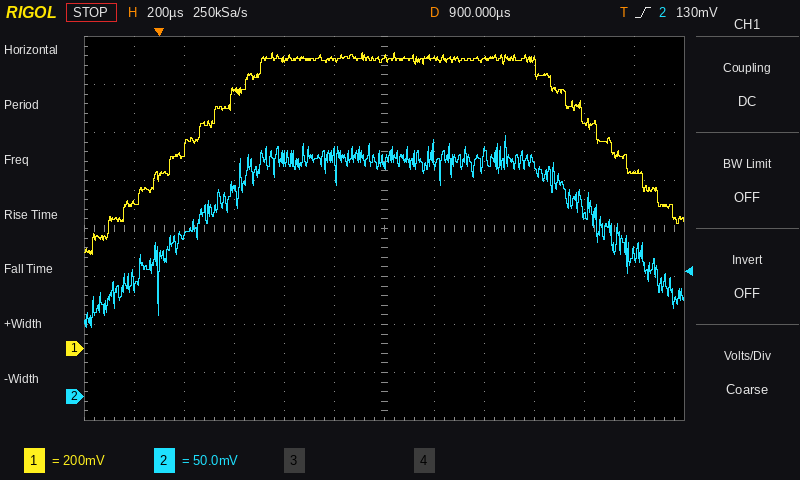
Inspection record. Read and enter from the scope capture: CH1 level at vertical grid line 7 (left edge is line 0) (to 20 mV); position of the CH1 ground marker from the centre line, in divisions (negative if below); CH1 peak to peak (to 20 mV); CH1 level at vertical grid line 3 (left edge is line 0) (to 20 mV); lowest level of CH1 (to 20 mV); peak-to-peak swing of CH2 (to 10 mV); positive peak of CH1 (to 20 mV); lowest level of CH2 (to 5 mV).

1.20 V
-2.5 div
840 mV
1.08 V
400 mV
200 mV
1.24 V
70 mV
